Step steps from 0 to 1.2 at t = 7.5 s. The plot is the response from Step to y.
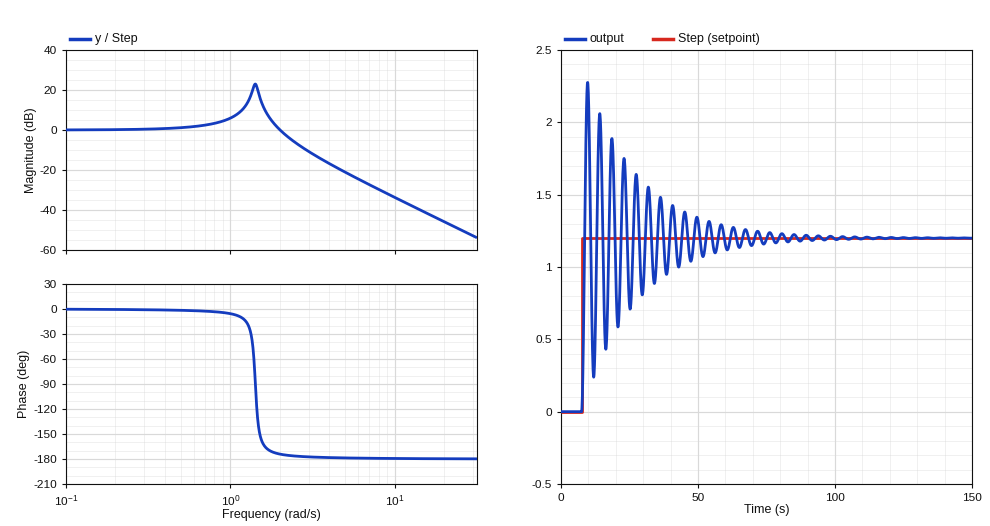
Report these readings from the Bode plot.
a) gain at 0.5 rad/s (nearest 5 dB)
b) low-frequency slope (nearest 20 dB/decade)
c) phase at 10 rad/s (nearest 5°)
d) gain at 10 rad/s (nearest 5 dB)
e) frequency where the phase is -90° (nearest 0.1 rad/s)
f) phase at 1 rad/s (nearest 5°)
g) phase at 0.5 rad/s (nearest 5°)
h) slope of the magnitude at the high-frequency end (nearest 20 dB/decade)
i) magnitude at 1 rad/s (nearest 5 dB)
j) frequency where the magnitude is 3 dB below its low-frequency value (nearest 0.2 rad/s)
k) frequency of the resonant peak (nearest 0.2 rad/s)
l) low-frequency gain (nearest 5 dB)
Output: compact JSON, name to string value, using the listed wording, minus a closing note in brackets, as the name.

{"gain at 0.5 rad/s": "0 dB", "low-frequency slope": "0 dB/decade", "phase at 10 rad/s": "-180°", "gain at 10 rad/s": "-35 dB", "frequency where the phase is -90°": "1.4 rad/s", "phase at 1 rad/s": "-5°", "phase at 0.5 rad/s": "0°", "slope of the magnitude at the high-frequency end": "-40 dB/decade", "magnitude at 1 rad/s": "5 dB", "frequency where the magnitude is 3 dB below its low-frequency value": "2.2 rad/s", "frequency of the resonant peak": "1.4 rad/s", "low-frequency gain": "0 dB"}
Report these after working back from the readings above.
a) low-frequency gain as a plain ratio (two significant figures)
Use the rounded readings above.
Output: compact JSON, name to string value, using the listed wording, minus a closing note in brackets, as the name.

{"low-frequency gain as a plain ratio": "1.0"}
